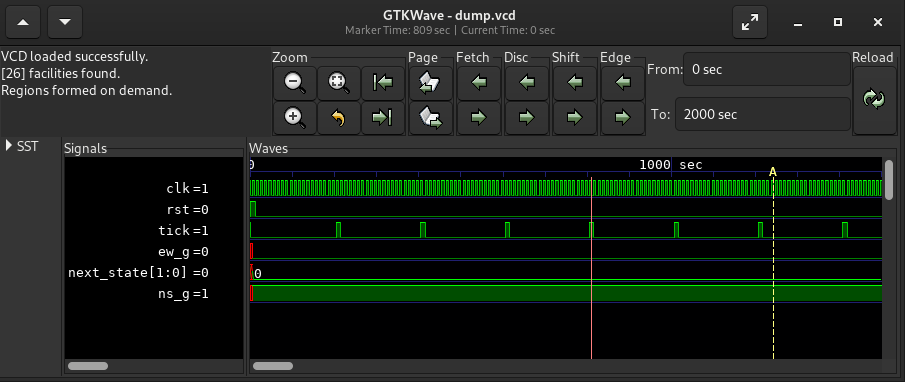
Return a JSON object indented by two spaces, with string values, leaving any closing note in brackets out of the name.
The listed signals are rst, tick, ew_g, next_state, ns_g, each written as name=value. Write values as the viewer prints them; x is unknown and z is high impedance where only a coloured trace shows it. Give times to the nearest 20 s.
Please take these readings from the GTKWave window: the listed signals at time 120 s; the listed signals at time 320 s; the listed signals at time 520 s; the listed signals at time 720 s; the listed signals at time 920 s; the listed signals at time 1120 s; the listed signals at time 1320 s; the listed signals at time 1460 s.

{
  "the listed signals at time 120 s": "rst=0, tick=0, ew_g=0, next_state=0, ns_g=1",
  "the listed signals at time 320 s": "rst=0, tick=0, ew_g=0, next_state=0, ns_g=1",
  "the listed signals at time 520 s": "rst=0, tick=0, ew_g=0, next_state=0, ns_g=1",
  "the listed signals at time 720 s": "rst=0, tick=0, ew_g=0, next_state=0, ns_g=1",
  "the listed signals at time 920 s": "rst=0, tick=0, ew_g=0, next_state=0, ns_g=1",
  "the listed signals at time 1120 s": "rst=0, tick=0, ew_g=0, next_state=0, ns_g=1",
  "the listed signals at time 1320 s": "rst=0, tick=0, ew_g=0, next_state=0, ns_g=1",
  "the listed signals at time 1460 s": "rst=0, tick=0, ew_g=0, next_state=0, ns_g=1"
}
